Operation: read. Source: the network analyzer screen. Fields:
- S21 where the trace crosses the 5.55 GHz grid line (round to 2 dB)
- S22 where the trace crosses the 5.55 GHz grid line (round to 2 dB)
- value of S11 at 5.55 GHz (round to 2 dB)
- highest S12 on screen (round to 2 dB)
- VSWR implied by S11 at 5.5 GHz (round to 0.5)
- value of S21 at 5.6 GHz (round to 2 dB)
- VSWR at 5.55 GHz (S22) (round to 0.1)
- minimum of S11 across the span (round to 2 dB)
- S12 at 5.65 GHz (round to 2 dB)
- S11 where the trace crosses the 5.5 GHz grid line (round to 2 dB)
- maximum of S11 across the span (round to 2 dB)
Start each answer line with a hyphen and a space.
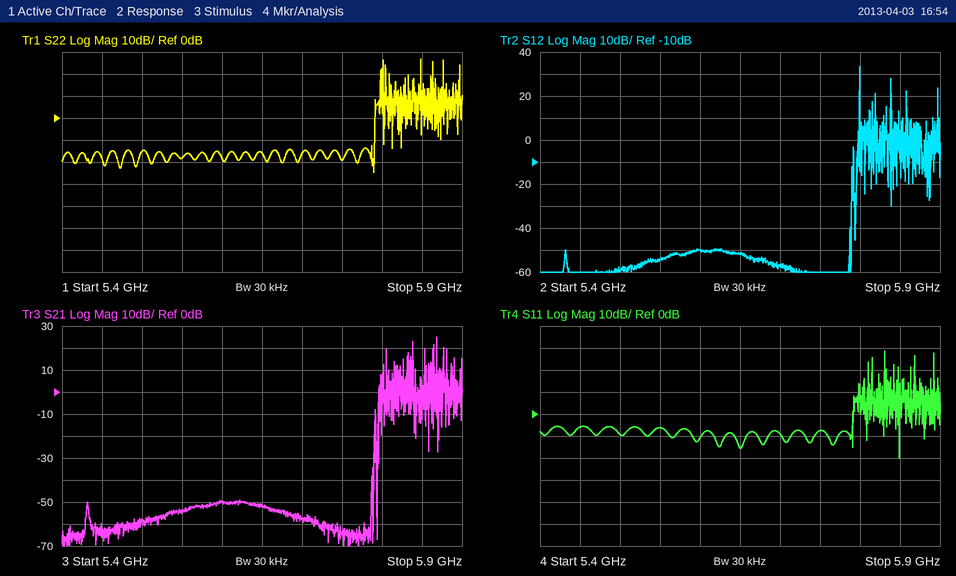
- -54 dB
- -18 dB
- -6 dB
- 34 dB
- 2.0
- -50 dB
- 1.3
- -20 dB
- -52 dB
- -10 dB
- 28 dB
